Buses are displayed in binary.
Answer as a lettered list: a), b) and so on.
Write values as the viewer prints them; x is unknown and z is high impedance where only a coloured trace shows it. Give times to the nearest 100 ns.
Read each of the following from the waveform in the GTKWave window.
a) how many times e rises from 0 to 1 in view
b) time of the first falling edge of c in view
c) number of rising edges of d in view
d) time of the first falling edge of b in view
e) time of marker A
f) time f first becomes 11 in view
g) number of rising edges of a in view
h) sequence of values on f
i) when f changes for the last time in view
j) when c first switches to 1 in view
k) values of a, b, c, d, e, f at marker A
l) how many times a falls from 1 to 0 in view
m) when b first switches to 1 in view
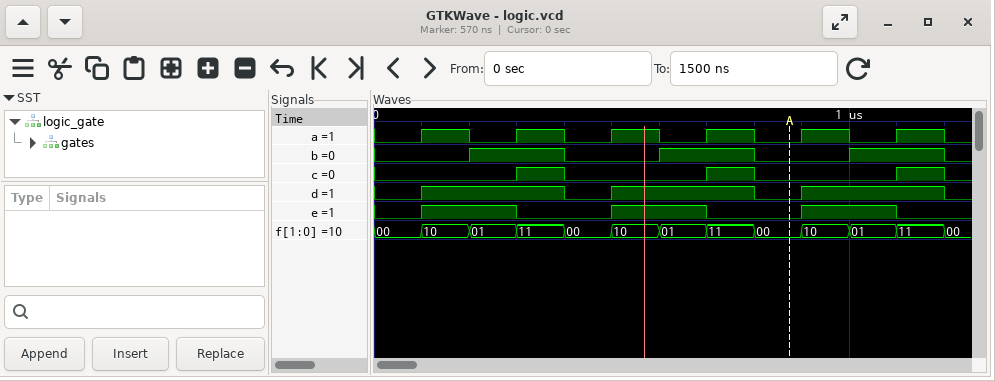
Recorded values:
a) 3
b) 400 ns
c) 3
d) 400 ns
e) 900 ns
f) 300 ns
g) 6
h) 00, 10, 01, 11, 00, 10, 01, 11, 00, 10, 01, 11, 00
i) 1200 ns
j) 300 ns
k) a=0, b=0, c=0, d=0, e=0, f=00
l) 6
m) 200 ns
